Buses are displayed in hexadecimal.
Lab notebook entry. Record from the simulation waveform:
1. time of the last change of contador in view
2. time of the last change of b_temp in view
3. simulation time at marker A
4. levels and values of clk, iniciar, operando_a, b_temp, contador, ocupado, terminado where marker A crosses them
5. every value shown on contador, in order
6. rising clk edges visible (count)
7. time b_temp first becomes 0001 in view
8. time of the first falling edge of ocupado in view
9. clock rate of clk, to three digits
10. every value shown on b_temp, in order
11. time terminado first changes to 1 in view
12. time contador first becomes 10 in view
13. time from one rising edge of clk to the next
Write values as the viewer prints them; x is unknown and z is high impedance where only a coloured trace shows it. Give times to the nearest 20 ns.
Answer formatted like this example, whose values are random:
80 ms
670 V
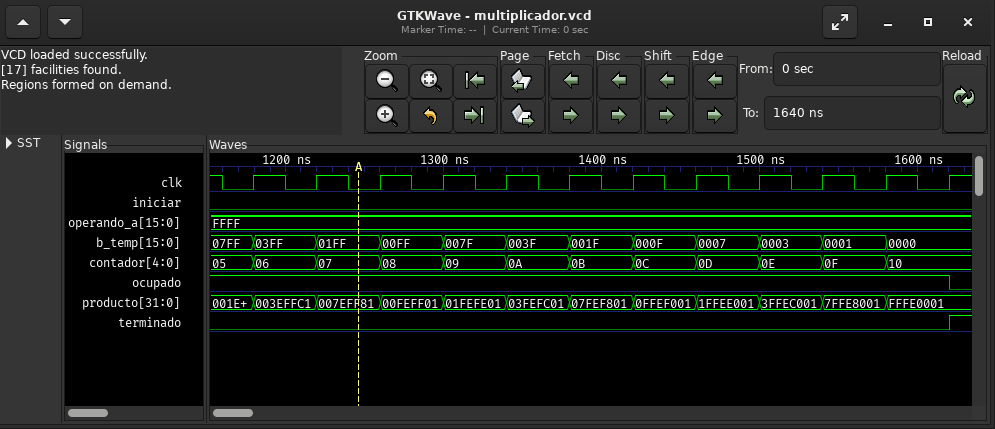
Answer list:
1580 ns
1580 ns
1240 ns
clk=0, iniciar=0, operando_a=FFFF, b_temp=01FF, contador=07, ocupado=1, terminado=0
05, 06, 07, 08, 09, 0A, 0B, 0C, 0D, 0E, 0F, 10
12
1540 ns
1620 ns
25.0 MHz
07FF, 03FF, 01FF, 00FF, 007F, 003F, 001F, 000F, 0007, 0003, 0001, 0000
1620 ns
1580 ns
40 ns
